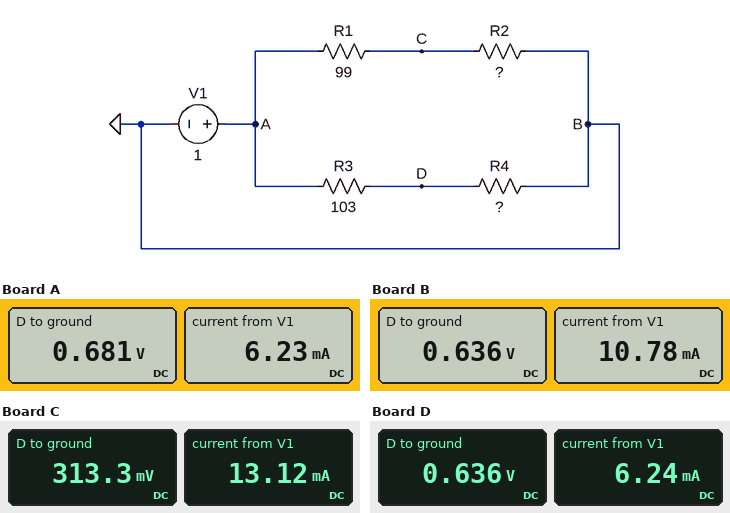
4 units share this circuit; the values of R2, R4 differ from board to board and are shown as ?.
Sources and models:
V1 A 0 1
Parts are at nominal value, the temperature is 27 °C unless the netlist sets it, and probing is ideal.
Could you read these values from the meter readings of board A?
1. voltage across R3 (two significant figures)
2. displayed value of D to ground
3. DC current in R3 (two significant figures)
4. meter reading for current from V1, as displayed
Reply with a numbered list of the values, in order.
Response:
1. 320 mV
2. 0.681 V
3. 3.1 mA
4. 6.23 mA
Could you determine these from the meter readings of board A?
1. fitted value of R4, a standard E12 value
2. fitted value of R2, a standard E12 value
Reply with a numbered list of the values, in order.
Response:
1. 220 Ω
2. 220 Ω
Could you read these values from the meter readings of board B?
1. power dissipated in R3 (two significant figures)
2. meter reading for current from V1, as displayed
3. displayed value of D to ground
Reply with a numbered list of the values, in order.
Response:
1. 1.3 mW
2. 10.78 mA
3. 0.636 V
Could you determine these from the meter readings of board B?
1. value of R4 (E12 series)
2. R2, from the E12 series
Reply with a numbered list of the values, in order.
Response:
1. 180 Ω
2. 39 Ω
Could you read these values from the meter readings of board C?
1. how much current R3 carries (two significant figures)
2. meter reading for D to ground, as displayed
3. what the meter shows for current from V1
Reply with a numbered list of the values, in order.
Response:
1. 6.7 mA
2. 313.3 mV
3. 13.12 mA
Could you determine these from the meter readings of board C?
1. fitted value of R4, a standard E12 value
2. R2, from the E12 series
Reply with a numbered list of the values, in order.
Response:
1. 47 Ω
2. 56 Ω
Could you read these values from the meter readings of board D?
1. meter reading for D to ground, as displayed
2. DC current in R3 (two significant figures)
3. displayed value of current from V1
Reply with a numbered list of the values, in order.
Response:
1. 0.636 V
2. 3.5 mA
3. 6.24 mA
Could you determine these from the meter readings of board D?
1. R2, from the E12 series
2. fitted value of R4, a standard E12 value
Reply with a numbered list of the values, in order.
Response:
1. 270 Ω
2. 180 Ω
